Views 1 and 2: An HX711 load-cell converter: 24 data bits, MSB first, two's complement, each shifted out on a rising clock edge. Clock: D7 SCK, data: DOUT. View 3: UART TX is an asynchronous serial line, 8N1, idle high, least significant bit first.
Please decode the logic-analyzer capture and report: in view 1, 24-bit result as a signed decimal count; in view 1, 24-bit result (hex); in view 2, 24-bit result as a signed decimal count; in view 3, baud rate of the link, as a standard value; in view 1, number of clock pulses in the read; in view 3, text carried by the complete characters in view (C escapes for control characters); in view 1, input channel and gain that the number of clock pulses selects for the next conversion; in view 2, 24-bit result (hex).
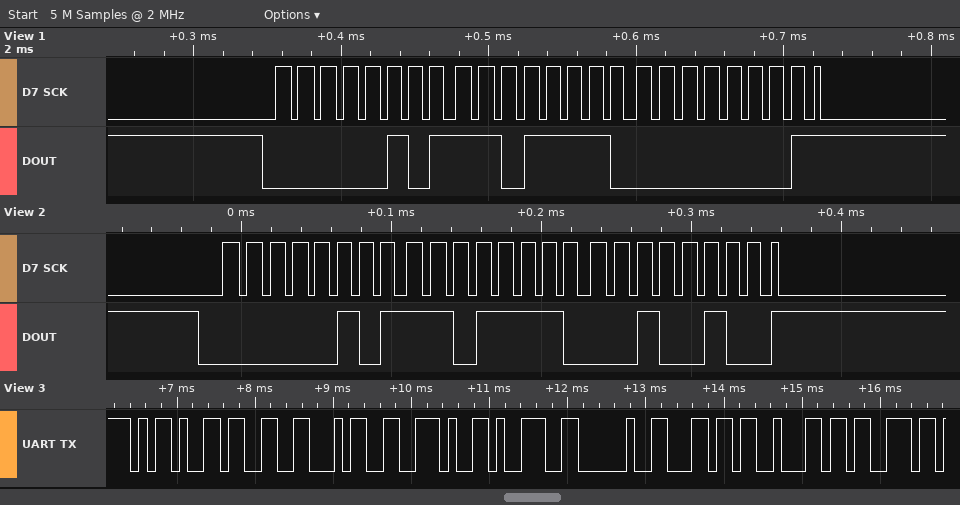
384513
0x05DE01
384548
9600 baud
25
"-34.9 lbs"
channel A, gain 128
0x05DE24
